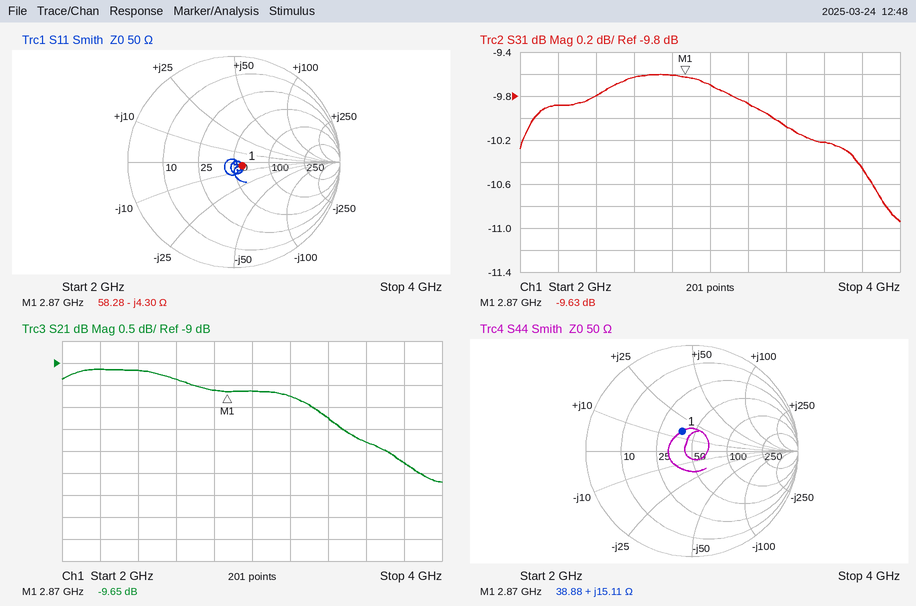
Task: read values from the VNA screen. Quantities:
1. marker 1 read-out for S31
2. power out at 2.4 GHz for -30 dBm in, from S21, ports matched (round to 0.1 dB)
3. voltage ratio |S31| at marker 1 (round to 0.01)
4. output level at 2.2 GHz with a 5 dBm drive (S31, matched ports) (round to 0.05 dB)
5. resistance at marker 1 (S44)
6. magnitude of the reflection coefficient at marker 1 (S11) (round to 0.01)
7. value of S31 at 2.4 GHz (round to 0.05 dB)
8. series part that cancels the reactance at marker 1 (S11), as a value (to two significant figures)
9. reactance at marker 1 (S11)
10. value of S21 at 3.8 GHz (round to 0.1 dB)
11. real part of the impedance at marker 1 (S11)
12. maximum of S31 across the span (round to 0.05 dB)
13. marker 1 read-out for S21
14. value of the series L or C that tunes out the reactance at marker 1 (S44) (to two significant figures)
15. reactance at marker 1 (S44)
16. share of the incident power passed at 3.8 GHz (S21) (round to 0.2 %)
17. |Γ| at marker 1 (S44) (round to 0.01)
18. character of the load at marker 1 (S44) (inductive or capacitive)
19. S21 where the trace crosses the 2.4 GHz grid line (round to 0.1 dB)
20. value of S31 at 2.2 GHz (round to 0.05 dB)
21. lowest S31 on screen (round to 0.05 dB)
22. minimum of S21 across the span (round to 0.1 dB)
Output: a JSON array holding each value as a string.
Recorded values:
["-9.63 dB", "-39.2 dBm", "0.33", "-4.90 dBm", "38.88 Ω", "0.09", "-9.80 dB", "240 pH", "-4.30 Ω", "-11.3 dB", "58.28 Ω", "-9.60 dB", "-9.65 dB", "3.7 pF", "+15.11 Ω", "7.4 %", "0.21", "inductive", "-9.2 dB", "-9.90 dB", "-10.95 dB", "-11.7 dB"]
